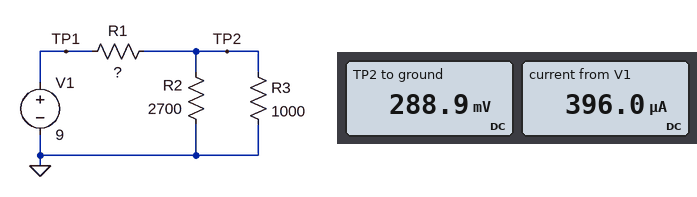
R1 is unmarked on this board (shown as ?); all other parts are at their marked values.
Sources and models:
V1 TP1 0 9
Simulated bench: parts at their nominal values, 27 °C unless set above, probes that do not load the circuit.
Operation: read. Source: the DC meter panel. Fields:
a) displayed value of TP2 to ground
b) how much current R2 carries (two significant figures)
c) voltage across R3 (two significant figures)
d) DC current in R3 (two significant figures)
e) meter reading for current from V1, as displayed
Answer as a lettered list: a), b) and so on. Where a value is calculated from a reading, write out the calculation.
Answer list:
a) 288.9 mV
b) (288.9 mV) / 2.7 kΩ = 110 µA
c) 288.9 mV = 290 mV
d) (288.9 mV) / 1 kΩ = 290 µA
e) 396.0 µA
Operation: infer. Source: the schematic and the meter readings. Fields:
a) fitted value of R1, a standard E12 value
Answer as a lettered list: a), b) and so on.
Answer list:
a) 22 kΩ
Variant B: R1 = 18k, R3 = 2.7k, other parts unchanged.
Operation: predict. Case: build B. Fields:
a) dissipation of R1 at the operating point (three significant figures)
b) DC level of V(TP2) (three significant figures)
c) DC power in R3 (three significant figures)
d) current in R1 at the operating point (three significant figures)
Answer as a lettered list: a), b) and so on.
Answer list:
a) 3.89 mW
b) 628 mV
c) 146 µW
d) 465 µA
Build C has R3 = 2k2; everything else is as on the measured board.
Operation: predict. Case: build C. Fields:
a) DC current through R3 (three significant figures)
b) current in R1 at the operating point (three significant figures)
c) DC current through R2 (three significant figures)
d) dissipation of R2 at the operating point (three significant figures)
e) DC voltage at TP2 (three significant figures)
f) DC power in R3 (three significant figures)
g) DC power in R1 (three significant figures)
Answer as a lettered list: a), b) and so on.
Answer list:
a) 214 µA
b) 388 µA
c) 174 µA
d) 81.8 µW
e) 470 mV
f) 100 µW
g) 3.31 mW
